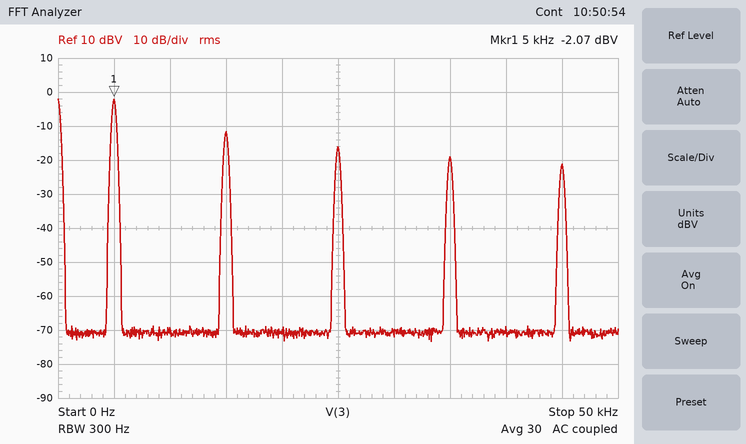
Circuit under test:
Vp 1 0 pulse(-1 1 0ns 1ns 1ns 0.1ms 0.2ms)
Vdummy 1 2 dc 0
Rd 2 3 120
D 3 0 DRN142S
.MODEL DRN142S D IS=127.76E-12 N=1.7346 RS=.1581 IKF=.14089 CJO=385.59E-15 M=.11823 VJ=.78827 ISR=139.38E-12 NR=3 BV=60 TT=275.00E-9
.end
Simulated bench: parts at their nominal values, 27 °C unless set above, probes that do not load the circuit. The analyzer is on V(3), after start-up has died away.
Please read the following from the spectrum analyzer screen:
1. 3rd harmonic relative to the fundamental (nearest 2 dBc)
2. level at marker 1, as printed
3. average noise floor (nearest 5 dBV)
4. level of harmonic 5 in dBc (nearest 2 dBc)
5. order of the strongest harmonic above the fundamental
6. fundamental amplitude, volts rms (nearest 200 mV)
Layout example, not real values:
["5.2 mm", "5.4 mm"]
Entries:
["-10 dBc", "-2.07 dBV", "-70 dBV", "-14 dBc", "3", "800 mV"]
